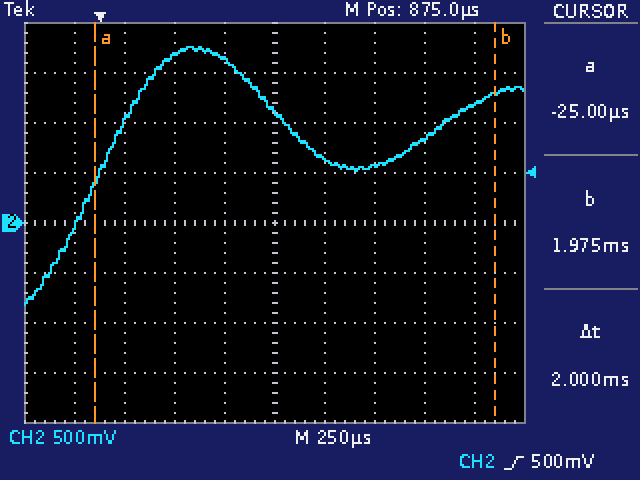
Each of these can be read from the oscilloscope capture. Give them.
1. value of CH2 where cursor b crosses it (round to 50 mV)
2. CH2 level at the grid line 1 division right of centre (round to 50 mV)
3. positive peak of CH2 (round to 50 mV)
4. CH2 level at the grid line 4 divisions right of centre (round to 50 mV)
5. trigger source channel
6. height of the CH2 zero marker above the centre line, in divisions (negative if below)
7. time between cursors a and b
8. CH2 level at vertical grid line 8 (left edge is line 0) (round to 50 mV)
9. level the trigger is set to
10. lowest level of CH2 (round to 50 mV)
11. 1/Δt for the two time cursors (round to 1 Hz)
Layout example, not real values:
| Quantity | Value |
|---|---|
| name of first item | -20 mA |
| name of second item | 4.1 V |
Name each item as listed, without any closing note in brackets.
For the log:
| Quantity | Value |
|---|---|
| value of CH2 where cursor b crosses it | 1.30 V |
| CH2 level at the grid line 1 division right of centre | 650 mV |
| positive peak of CH2 | 1.75 V |
| CH2 level at the grid line 4 divisions right of centre | 1.20 V |
| trigger source channel | CH2 |
| height of the CH2 zero marker above the centre line, in divisions | 0.0 div |
| time between cursors a and b | 2 ms |
| CH2 level at vertical grid line 8 (left edge is line 0) | 850 mV |
| level the trigger is set to | 500 mV |
| lowest level of CH2 | -800 mV |
| 1/Δt for the two time cursors | 500 Hz |
